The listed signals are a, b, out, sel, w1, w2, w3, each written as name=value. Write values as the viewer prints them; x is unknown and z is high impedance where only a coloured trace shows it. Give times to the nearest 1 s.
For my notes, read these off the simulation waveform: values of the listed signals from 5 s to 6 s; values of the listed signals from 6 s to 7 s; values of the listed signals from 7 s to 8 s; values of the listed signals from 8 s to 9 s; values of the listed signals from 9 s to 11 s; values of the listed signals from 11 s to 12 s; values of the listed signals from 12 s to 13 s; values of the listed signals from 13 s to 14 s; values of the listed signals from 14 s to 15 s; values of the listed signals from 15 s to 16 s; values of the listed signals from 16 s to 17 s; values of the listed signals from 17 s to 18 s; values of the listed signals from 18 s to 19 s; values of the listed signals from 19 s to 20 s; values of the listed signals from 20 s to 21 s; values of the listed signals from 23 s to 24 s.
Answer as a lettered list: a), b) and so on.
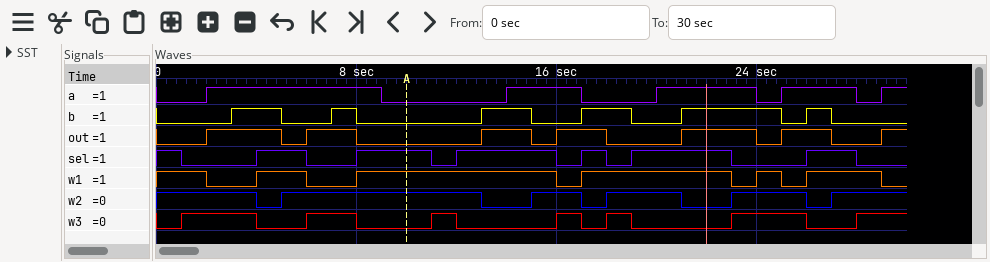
a) a=1, b=0, out=0, sel=1, w1=1, w2=1, w3=0
b) a=1, b=0, out=1, sel=0, w1=0, w2=1, w3=1
c) a=1, b=1, out=1, sel=0, w1=0, w2=1, w3=1
d) a=1, b=0, out=0, sel=1, w1=1, w2=1, w3=0
e) a=0, b=0, out=0, sel=1, w1=1, w2=1, w3=0
f) a=0, b=0, out=0, sel=0, w1=1, w2=1, w3=1
g) a=0, b=0, out=0, sel=1, w1=1, w2=1, w3=0
h) a=0, b=1, out=1, sel=1, w1=1, w2=0, w3=0
i) a=1, b=1, out=1, sel=1, w1=1, w2=0, w3=0
j) a=1, b=0, out=0, sel=1, w1=1, w2=1, w3=0
k) a=1, b=0, out=1, sel=0, w1=0, w2=1, w3=1
l) a=0, b=1, out=1, sel=1, w1=1, w2=0, w3=0
m) a=0, b=1, out=0, sel=0, w1=1, w2=1, w3=1
n) a=0, b=0, out=0, sel=1, w1=1, w2=1, w3=0
o) a=1, b=0, out=0, sel=1, w1=1, w2=1, w3=0
p) a=1, b=1, out=1, sel=0, w1=0, w2=1, w3=1
